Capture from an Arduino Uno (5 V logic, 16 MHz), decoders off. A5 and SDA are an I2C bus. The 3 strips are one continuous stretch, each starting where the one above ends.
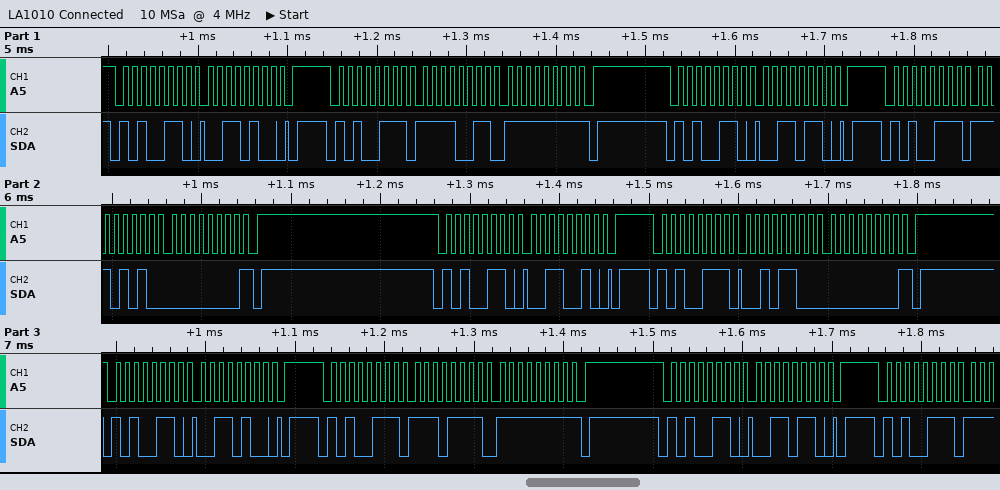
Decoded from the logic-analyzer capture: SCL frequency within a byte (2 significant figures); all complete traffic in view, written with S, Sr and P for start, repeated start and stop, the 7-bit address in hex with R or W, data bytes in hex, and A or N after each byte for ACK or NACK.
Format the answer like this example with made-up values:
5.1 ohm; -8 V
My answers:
100 kHz; S 53W A 34 A P S 53R A F3 A FF N P S 53W A 36 A P S 53R A EA A 00 N P S 53W A 32 A P S 53R A 2C A 00 N P S 53W A 34 A P S 53R A EF A FF N P S 53W A 36 A P S 53R A
